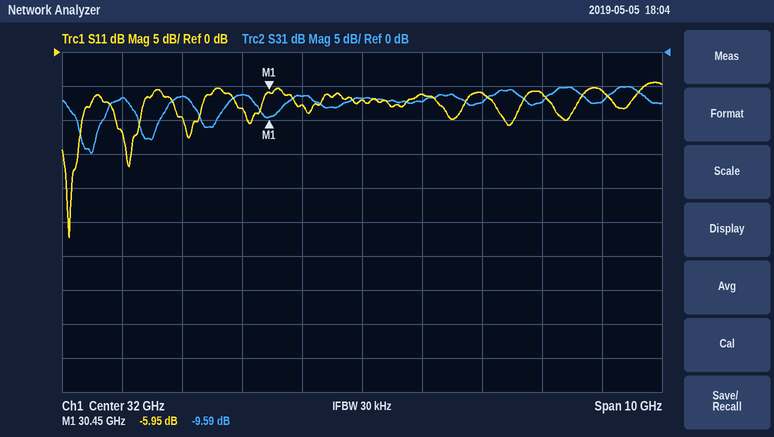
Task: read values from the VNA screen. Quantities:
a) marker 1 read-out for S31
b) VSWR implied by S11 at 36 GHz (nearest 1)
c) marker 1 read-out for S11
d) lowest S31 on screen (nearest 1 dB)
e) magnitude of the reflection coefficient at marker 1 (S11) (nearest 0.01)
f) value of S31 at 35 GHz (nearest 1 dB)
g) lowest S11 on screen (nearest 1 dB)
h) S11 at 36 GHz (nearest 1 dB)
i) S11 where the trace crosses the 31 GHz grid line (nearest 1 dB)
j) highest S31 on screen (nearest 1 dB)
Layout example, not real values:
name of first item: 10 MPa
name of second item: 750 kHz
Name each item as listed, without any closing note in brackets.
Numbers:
marker 1 read-out for S31: -9.59 dB
VSWR implied by S11 at 36 GHz: 3
marker 1 read-out for S11: -5.95 dB
lowest S31 on screen: -15 dB
magnitude of the reflection coefficient at marker 1 (S11): 0.50
value of S31 at 35 GHz: -7 dB
lowest S11 on screen: -27 dB
S11 at 36 GHz: -6 dB
S11 where the trace crosses the 31 GHz grid line: -8 dB
highest S31 on screen: -5 dB
